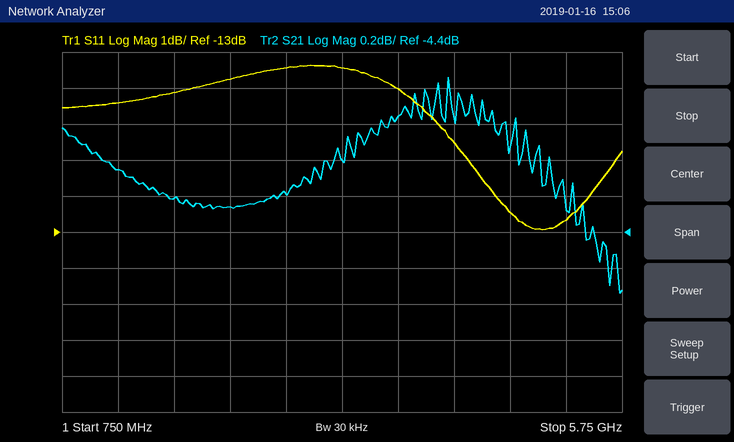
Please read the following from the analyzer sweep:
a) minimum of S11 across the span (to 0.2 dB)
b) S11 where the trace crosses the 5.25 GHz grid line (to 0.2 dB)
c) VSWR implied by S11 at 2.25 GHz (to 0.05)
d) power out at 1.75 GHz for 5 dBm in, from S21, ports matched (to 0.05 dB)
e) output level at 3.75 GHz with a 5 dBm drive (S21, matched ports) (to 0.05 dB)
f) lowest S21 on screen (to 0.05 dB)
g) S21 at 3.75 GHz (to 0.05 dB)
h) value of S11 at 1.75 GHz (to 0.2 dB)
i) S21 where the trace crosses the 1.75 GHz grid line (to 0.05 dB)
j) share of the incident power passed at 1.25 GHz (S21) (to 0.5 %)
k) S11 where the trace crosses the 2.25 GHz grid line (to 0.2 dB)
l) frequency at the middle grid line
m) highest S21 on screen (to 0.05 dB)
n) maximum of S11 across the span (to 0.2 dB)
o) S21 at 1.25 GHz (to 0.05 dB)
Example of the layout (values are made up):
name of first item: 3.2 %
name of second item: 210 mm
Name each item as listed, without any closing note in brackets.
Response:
minimum of S11 across the span: -13.0 dB
S11 where the trace crosses the 5.25 GHz grid line: -12.6 dB
VSWR implied by S11 at 2.25 GHz: 2.15
power out at 1.75 GHz for 5 dBm in, from S21, ports matched: 0.80 dBm
output level at 3.75 GHz with a 5 dBm drive (S21, matched ports): 1.25 dBm
lowest S21 on screen: -4.75 dB
S21 at 3.75 GHz: -3.75 dB
value of S11 at 1.75 GHz: -9.2 dB
S21 where the trace crosses the 1.75 GHz grid line: -4.20 dB
share of the incident power passed at 1.25 GHz (S21): 39.5 %
S11 where the trace crosses the 2.25 GHz grid line: -8.8 dB
frequency at the middle grid line: 3.25 GHz
highest S21 on screen: -3.55 dB
maximum of S11 across the span: -8.4 dB
S21 at 1.25 GHz: -4.05 dB
